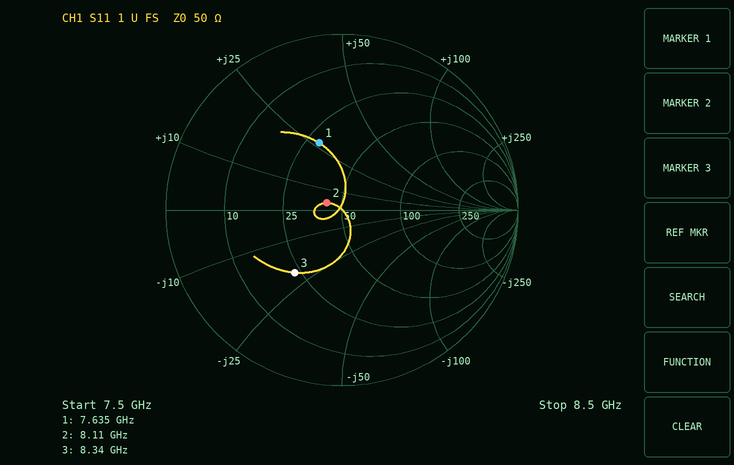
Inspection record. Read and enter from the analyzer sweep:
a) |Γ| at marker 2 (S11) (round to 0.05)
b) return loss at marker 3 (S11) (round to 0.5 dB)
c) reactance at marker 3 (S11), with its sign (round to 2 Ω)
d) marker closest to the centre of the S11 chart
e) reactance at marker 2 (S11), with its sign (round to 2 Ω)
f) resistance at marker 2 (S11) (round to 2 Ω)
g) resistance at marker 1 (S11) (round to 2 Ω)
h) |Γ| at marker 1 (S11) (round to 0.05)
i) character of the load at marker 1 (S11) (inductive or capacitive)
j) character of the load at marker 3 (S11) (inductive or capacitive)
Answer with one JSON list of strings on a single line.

["0.10", "7.0 dB", "-20 Ω", "marker 2", "+4 Ω", "42 Ω", "30 Ω", "0.40", "inductive", "capacitive"]
